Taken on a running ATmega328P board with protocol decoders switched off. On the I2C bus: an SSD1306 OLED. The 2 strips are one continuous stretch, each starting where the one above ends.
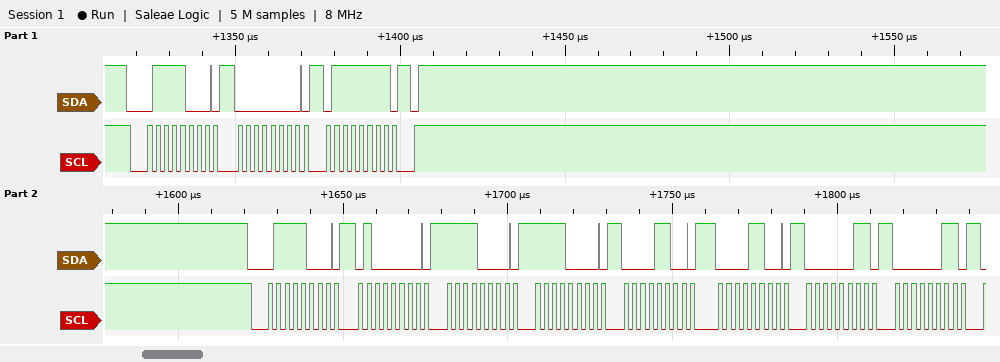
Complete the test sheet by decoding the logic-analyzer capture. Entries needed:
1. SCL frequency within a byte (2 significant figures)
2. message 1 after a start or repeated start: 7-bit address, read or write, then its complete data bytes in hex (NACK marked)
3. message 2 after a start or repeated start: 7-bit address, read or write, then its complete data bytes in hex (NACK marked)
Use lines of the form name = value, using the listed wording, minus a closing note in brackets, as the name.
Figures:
SCL frequency within a byte = 400 kHz
message 1 after a start or repeated start: 7-bit address, read or write, then its complete data bytes in hex = 0x3C write: 00 7F
message 2 after a start or repeated start: 7-bit address, read or write, then its complete data bytes in hex = 0x3C write: 40 F0 F0 0C 0C 03 03
